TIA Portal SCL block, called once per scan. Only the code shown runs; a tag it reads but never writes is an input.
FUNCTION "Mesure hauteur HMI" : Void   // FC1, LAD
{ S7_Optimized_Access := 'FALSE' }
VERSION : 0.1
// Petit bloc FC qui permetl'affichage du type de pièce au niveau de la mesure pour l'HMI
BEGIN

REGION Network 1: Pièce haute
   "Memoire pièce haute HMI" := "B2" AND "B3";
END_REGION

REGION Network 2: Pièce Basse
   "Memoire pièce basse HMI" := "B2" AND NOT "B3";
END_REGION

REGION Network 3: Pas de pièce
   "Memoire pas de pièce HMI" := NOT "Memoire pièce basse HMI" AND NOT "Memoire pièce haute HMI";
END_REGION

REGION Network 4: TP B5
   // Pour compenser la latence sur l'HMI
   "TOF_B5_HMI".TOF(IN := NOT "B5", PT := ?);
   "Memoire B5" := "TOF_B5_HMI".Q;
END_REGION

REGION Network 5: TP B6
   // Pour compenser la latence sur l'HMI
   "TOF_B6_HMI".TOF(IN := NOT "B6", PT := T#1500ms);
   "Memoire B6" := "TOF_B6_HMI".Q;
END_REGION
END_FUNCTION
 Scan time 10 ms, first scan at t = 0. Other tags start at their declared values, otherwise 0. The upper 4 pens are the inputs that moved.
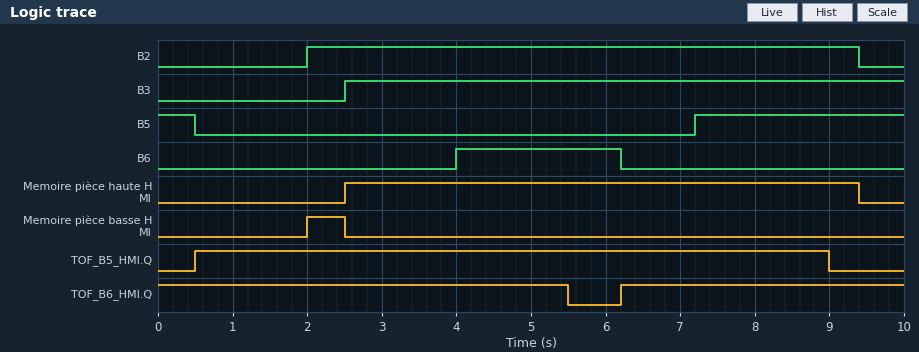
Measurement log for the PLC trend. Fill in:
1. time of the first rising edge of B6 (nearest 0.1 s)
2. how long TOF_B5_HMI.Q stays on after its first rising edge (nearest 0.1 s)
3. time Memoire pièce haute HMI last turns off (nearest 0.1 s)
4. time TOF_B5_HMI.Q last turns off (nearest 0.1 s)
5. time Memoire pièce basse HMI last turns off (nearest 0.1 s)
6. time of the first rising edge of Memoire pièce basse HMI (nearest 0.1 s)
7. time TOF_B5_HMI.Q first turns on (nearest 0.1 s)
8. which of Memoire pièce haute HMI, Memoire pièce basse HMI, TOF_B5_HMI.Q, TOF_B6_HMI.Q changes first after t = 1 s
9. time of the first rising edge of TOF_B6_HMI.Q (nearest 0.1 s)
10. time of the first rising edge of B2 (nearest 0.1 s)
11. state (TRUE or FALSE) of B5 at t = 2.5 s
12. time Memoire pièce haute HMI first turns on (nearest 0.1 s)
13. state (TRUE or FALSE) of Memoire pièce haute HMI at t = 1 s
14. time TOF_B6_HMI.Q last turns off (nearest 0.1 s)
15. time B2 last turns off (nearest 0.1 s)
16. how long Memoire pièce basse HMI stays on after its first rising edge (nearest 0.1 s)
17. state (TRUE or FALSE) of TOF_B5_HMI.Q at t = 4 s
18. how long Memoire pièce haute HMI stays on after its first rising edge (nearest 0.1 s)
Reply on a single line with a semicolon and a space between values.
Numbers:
4.0 s; 8.5 s; 9.4 s; 9.0 s; 2.5 s; 2.0 s; 0.5 s; Memoire pièce basse HMI; 6.2 s; 2.0 s; FALSE; 2.5 s; FALSE; 5.5 s; 9.4 s; 0.5 s; TRUE; 6.9 s
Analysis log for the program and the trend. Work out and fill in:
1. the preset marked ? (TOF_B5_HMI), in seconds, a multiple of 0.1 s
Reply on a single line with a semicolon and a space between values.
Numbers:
1.8 s
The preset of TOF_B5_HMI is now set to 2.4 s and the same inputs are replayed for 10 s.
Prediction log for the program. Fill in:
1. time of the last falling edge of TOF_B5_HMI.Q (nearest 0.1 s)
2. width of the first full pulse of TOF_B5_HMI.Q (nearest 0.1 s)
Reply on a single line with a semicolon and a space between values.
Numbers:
9.6 s; 9.1 s
